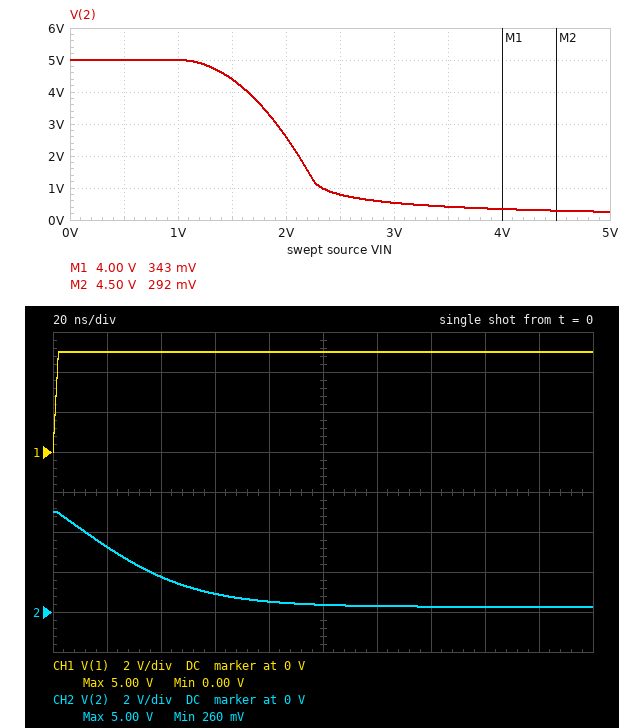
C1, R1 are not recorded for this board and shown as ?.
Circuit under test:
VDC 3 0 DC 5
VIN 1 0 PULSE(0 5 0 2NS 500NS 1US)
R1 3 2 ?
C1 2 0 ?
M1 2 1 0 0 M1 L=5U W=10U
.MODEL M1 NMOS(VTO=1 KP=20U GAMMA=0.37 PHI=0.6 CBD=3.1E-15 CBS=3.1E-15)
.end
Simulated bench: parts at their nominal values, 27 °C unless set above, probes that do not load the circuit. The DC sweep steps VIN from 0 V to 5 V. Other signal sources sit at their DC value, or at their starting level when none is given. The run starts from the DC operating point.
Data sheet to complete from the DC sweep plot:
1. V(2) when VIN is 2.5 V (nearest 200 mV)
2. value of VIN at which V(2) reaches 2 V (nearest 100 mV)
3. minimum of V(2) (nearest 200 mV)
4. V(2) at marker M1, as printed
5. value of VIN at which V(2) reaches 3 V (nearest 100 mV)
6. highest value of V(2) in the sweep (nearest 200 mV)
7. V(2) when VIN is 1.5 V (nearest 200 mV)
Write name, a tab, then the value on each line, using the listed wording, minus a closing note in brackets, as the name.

V(2) when VIN is 2.5 V	800 mV
value of VIN at which V(2) reaches 2 V	2.1 V
minimum of V(2)	200 mV
V(2) at marker M1, as printed	343 mV
value of VIN at which V(2) reaches 3 V	1.9 V
highest value of V(2) in the sweep	5.0 V
V(2) when VIN is 1.5 V	4.4 V
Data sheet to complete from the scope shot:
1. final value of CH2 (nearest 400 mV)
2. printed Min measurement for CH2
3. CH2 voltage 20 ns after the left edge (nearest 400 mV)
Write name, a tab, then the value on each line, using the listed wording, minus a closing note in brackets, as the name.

final value of CH2	400 mV
printed Min measurement for CH2	260 mV
CH2 voltage 20 ns after the left edge	3.2 V
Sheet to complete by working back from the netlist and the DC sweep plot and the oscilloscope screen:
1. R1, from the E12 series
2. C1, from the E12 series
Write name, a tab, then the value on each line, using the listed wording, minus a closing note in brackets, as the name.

R1, from the E12 series	120 kΩ
C1, from the E12 series	3.3 pF
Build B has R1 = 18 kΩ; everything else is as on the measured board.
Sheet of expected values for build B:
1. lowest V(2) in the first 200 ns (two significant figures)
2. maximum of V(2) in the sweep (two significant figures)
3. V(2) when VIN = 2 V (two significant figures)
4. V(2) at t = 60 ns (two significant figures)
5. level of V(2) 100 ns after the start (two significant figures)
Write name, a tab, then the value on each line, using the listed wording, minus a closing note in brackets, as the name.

lowest V(2) in the first 200 ns	1.5 V
maximum of V(2) in the sweep	5.0 V
V(2) when VIN = 2 V	4.6 V
V(2) at t = 60 ns	1.9 V
level of V(2) 100 ns after the start	1.6 V
